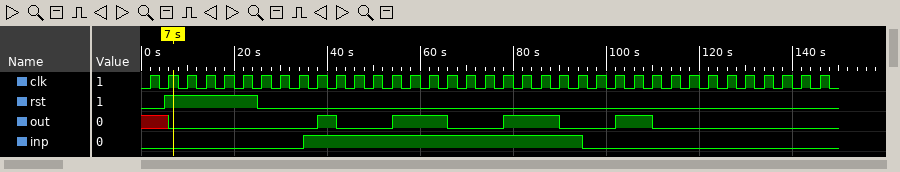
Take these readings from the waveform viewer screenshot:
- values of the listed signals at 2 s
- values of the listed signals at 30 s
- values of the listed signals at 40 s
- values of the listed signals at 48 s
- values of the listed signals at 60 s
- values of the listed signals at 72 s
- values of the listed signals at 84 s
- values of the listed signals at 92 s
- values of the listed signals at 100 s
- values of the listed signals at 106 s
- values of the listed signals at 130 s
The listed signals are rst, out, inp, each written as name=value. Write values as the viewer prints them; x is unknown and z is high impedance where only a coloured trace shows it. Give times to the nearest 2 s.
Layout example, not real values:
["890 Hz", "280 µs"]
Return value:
["rst=0, out=x, inp=0", "rst=0, out=0, inp=0", "rst=0, out=1, inp=1", "rst=0, out=0, inp=1", "rst=0, out=1, inp=1", "rst=0, out=0, inp=1", "rst=0, out=1, inp=1", "rst=0, out=0, inp=1", "rst=0, out=0, inp=0", "rst=0, out=1, inp=0", "rst=0, out=0, inp=0"]
